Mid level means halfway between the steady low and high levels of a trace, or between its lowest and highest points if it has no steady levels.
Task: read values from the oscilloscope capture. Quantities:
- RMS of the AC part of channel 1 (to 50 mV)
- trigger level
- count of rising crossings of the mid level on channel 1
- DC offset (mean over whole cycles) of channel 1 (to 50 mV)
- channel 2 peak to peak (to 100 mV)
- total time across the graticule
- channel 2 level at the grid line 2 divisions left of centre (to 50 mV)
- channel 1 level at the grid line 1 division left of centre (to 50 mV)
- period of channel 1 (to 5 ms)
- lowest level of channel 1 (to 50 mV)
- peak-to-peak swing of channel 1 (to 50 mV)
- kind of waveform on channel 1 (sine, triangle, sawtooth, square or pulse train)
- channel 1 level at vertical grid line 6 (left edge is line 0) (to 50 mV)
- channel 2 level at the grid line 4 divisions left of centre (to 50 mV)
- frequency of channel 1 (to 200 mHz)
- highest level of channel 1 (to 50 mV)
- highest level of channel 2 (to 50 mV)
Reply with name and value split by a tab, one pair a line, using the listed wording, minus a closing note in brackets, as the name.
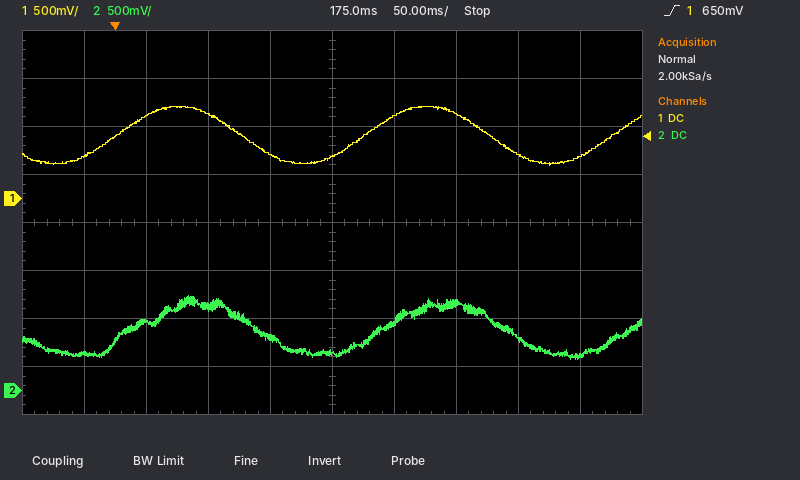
RMS of the AC part of channel 1	200 mV
trigger level	650 mV
count of rising crossings of the mid level on channel 1	3
DC offset (mean over whole cycles) of channel 1	650 mV
channel 2 peak to peak	700 mV
total time across the graticule	500 ms
channel 2 level at the grid line 2 divisions left of centre	850 mV
channel 1 level at the grid line 1 division left of centre	450 mV
period of channel 1	200 ms
lowest level of channel 1	350 mV
peak-to-peak swing of channel 1	600 mV
kind of waveform on channel 1	sine
channel 1 level at vertical grid line 6 (left edge is line 0)	850 mV
channel 2 level at the grid line 4 divisions left of centre	400 mV
frequency of channel 1	5.0 Hz
highest level of channel 1	950 mV
highest level of channel 2	1.00 V
